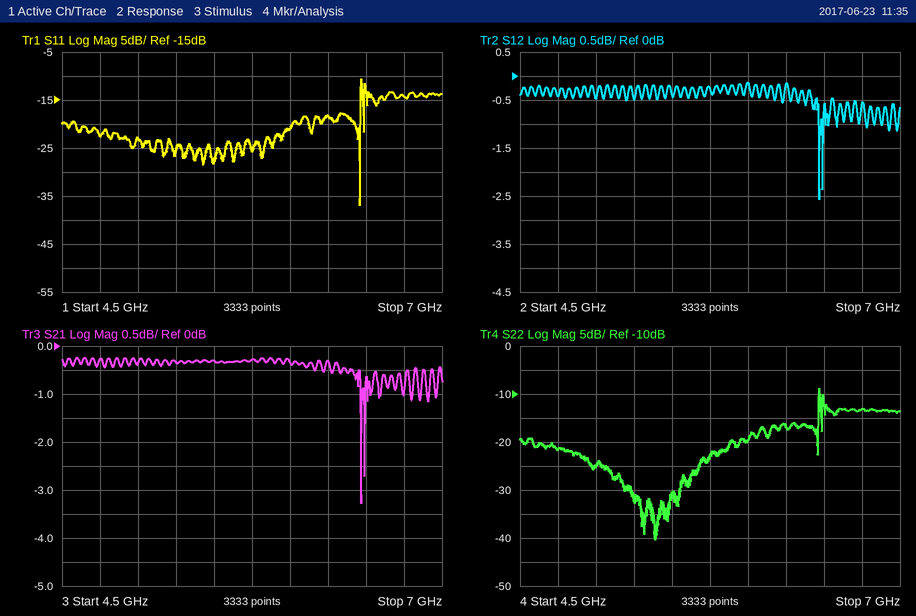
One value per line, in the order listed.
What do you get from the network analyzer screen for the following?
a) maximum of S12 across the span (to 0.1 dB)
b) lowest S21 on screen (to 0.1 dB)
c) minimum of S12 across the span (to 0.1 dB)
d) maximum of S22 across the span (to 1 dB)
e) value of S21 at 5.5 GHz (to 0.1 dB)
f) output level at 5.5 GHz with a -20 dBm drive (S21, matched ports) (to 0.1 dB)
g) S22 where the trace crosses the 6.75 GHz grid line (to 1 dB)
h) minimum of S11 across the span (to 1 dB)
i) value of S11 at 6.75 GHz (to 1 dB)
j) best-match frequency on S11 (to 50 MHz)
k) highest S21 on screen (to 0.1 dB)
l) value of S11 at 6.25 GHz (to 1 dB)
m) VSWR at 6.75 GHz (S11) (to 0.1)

-0.1 dB
-3.3 dB
-2.6 dB
-9 dB
-0.3 dB
-20.3 dBm
-13 dB
-37 dB
-14 dB
6.45 GHz
-0.2 dB
-18 dB
1.5
